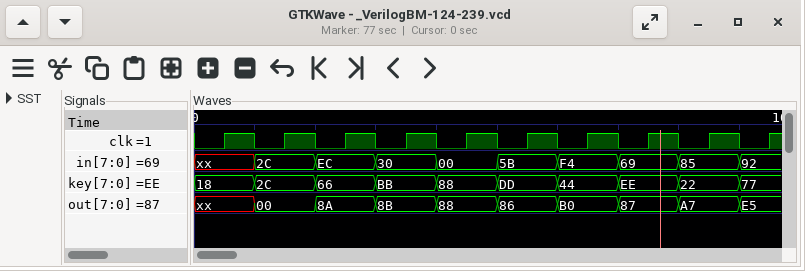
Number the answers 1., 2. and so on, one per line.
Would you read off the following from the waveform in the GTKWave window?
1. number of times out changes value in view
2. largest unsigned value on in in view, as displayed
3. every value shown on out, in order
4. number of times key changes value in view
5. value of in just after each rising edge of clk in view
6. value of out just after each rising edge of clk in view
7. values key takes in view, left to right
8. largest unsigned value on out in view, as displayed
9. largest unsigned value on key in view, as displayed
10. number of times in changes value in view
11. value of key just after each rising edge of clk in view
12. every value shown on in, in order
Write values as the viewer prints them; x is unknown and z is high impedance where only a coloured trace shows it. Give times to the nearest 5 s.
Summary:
1. 9
2. F4
3. xx, 00, 8A, 8B, 88, 86, B0, 87, A7, E5
4. 9
5. xx, 2C, EC, 30, 00, 5B, F4, 69, 85, 92
6. xx, 00, 8A, 8B, 88, 86, B0, 87, A7, E5
7. 18, 2C, 66, BB, 88, DD, 44, EE, 22, 77
8. E5
9. EE
10. 9
11. 18, 2C, 66, BB, 88, DD, 44, EE, 22, 77
12. xx, 2C, EC, 30, 00, 5B, F4, 69, 85, 92
